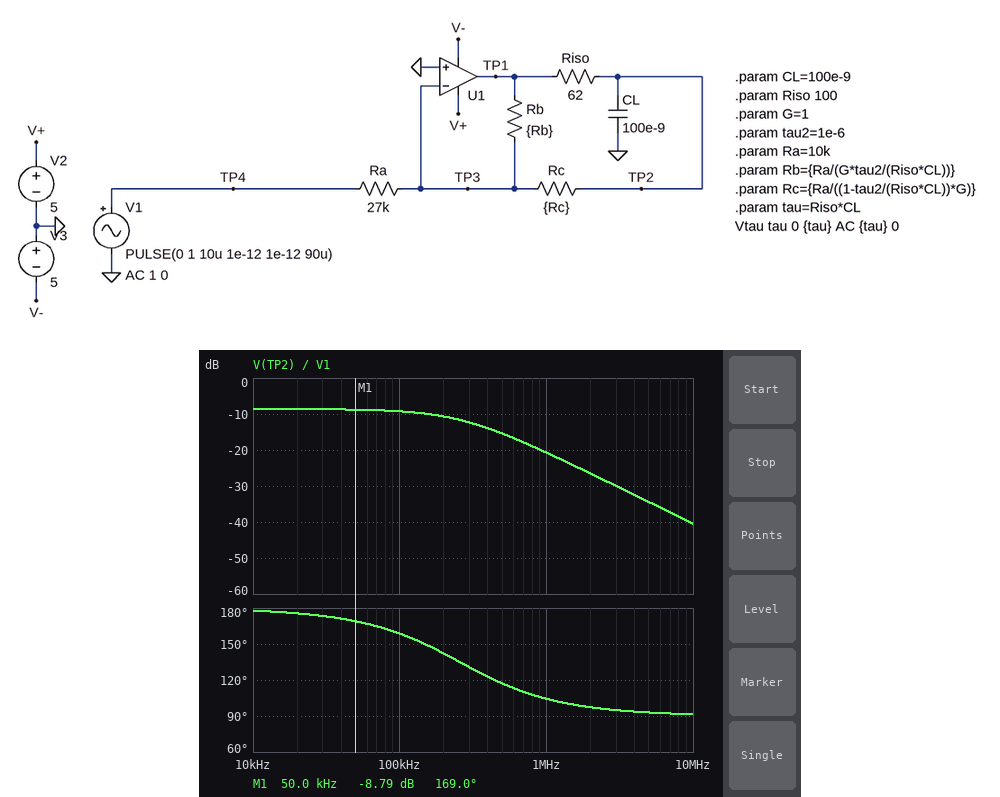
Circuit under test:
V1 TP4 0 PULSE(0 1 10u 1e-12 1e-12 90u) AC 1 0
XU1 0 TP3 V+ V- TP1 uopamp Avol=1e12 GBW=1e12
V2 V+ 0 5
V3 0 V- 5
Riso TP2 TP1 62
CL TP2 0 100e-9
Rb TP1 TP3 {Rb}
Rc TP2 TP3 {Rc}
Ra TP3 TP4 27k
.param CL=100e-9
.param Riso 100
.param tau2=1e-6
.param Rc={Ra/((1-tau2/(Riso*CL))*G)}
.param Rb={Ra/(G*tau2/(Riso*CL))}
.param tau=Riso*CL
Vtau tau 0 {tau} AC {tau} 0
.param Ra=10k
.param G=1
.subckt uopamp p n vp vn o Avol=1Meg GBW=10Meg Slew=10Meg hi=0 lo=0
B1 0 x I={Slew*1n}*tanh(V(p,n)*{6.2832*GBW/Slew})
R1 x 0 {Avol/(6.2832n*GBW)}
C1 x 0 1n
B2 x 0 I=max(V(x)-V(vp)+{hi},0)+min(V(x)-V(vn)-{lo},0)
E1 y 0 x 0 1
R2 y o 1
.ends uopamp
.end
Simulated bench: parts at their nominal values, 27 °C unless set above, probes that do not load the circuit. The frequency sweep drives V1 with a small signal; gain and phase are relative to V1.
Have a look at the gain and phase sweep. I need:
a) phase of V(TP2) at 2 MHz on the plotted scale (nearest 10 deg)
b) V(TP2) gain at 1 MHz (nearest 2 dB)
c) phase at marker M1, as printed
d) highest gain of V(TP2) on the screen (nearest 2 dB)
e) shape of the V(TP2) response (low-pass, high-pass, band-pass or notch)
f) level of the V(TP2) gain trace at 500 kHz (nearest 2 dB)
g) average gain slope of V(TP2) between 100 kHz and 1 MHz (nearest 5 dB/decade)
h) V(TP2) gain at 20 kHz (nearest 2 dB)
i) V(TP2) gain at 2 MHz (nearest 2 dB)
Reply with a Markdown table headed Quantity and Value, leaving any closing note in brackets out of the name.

| Quantity | Value |
|---|---|
| phase of V(TP2) at 2 MHz on the plotted scale | 100 deg |
| V(TP2) gain at 1 MHz | -20 dB |
| phase at marker M1, as printed | 169.0 deg |
| highest gain of V(TP2) on the screen | -8 dB |
| shape of the V(TP2) response | low-pass |
| level of the V(TP2) gain trace at 500 kHz | -16 dB |
| average gain slope of V(TP2) between 100 kHz and 1 MHz | -10 dB/decade |
| V(TP2) gain at 20 kHz | -8 dB |
| V(TP2) gain at 2 MHz | -26 dB |
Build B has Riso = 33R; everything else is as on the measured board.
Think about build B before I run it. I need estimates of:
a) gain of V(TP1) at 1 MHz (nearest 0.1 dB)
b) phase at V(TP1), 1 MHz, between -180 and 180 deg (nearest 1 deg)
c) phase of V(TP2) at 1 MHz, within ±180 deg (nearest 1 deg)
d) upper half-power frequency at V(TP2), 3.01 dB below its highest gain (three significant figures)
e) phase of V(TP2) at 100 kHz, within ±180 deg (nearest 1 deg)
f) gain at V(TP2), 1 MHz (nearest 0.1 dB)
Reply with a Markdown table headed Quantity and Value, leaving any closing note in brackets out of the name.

| Quantity | Value |
|---|---|
| gain of V(TP1) at 1 MHz | 10.5 dB |
| phase at V(TP1), 1 MHz, between -180 and 180 deg | -157 deg |
| phase of V(TP2) at 1 MHz, within ±180 deg | 116 deg |
| upper half-power frequency at V(TP2), 3.01 dB below its highest gain | 482 kHz |
| phase of V(TP2) at 100 kHz, within ±180 deg | 168 deg |
| gain at V(TP2), 1 MHz | -15.9 dB |
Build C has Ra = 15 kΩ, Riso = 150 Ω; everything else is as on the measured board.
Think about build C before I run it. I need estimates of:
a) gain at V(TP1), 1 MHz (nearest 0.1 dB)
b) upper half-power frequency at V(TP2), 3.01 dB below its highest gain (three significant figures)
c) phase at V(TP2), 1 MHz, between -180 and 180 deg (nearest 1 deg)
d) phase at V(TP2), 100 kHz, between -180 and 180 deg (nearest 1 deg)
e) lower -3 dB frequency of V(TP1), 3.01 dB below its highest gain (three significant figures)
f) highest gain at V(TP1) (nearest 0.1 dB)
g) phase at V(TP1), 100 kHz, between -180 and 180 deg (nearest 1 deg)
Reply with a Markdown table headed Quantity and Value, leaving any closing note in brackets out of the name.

| Quantity | Value |
|---|---|
| gain at V(TP1), 1 MHz | 16.4 dB |
| upper half-power frequency at V(TP2), 3.01 dB below its highest gain | 106 kHz |
| phase at V(TP2), 1 MHz, between -180 and 180 deg | 96 deg |
| phase at V(TP2), 100 kHz, between -180 and 180 deg | 137 deg |
| lower -3 dB frequency of V(TP1), 3.01 dB below its highest gain | 105 kHz |
| highest gain at V(TP1) | 16.5 dB |
| phase at V(TP1), 100 kHz, between -180 and 180 deg | -139 deg |
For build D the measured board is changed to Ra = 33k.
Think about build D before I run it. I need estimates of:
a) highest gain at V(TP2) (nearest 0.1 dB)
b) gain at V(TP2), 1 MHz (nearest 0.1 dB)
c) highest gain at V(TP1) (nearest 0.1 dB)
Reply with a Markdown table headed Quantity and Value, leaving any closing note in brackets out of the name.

| Quantity | Value |
|---|---|
| highest gain at V(TP2) | -10.4 dB |
| gain at V(TP2), 1 MHz | -22.5 dB |
| highest gain at V(TP1) | 9.6 dB |
